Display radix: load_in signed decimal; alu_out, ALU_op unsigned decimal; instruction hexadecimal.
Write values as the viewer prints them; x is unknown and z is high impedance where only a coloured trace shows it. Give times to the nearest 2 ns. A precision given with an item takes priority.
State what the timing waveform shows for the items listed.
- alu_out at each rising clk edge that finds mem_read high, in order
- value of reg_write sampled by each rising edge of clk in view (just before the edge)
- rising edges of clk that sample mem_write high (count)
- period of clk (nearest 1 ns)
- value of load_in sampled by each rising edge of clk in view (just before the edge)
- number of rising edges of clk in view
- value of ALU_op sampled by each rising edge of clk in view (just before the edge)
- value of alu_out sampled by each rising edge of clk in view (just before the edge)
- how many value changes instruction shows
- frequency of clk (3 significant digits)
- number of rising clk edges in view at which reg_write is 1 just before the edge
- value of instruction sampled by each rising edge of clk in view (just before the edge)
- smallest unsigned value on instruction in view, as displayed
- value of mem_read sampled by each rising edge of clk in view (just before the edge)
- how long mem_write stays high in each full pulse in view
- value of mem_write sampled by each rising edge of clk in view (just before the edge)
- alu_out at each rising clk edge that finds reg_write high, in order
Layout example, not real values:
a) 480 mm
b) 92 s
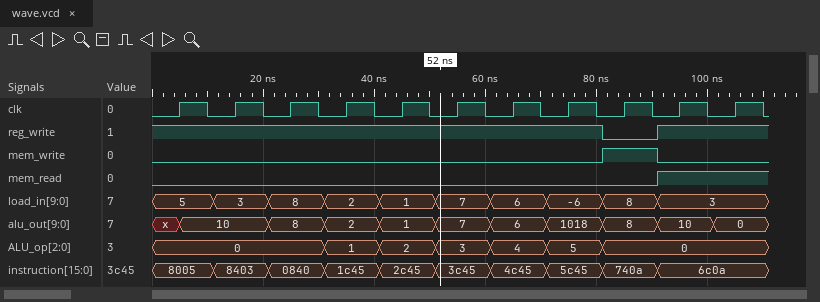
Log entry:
a) 10, 0
b) 1 1 1 1 1 1 1 1 0 1 1
c) 1
d) 10 ns
e) 5, 3, 8, 2, 1, 7, 6, -6, 8, 3, 3
f) 11
g) 0, 0, 0, 1, 2, 3, 4, 5, 0, 0, 0
h) x, 10, 8, 2, 1, 7, 6, 1018, 8, 10, 0
i) 9
j) 100 MHz
k) 10
l) 8005, 8403, 0840, 1c45, 2c45, 3c45, 4c45, 5c45, 740a, 6c0a, 6c0a
m) 0840
n) 0 0 0 0 0 0 0 0 0 1 1
o) 10 ns
p) 0 0 0 0 0 0 0 0 1 0 0
q) x, 10, 8, 2, 1, 7, 6, 1018, 10, 0
